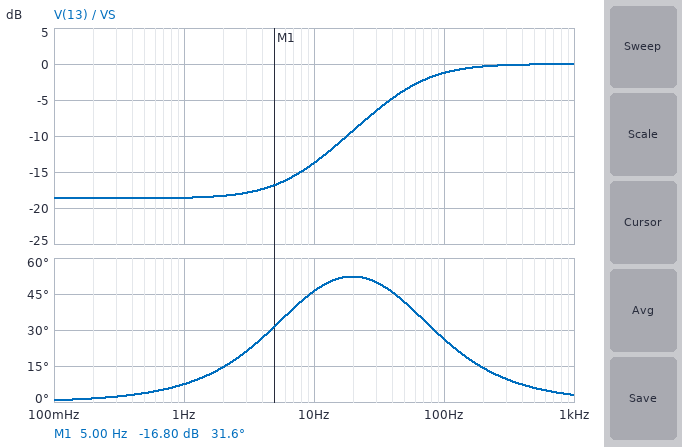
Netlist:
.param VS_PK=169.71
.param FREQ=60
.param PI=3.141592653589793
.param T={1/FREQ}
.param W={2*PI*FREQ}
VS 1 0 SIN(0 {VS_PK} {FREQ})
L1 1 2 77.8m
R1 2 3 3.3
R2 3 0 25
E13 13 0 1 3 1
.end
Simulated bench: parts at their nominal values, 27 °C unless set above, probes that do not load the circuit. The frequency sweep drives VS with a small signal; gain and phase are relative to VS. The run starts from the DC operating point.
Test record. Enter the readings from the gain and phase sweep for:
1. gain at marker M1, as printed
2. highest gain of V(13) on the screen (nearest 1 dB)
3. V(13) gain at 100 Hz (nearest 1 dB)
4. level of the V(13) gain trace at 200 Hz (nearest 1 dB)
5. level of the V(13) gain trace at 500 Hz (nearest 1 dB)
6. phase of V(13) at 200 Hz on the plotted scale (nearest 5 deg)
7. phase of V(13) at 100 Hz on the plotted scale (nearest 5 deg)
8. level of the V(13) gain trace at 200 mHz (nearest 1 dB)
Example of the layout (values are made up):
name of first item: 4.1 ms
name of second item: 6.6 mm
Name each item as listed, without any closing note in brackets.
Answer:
gain at marker M1, as printed: -16.80 dB
highest gain of V(13) on the screen: 0 dB
V(13) gain at 100 Hz: -1 dB
level of the V(13) gain trace at 200 Hz: 0 dB
level of the V(13) gain trace at 500 Hz: 0 dB
phase of V(13) at 200 Hz on the plotted scale: 15 deg
phase of V(13) at 100 Hz on the plotted scale: 25 deg
level of the V(13) gain trace at 200 mHz: -19 dB
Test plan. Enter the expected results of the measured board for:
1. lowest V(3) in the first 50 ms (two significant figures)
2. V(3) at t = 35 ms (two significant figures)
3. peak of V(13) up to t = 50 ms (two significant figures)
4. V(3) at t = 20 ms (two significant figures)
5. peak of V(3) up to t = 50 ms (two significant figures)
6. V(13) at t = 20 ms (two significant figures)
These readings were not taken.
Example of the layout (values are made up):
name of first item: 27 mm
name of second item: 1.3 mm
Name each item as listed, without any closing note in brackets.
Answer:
lowest V(3) in the first 50 ms: -100 V
V(3) at t = 35 ms: -18 V
peak of V(13) up to t = 50 ms: 120 V
V(3) at t = 20 ms: 46 V
peak of V(3) up to t = 50 ms: 110 V
V(13) at t = 20 ms: 120 V
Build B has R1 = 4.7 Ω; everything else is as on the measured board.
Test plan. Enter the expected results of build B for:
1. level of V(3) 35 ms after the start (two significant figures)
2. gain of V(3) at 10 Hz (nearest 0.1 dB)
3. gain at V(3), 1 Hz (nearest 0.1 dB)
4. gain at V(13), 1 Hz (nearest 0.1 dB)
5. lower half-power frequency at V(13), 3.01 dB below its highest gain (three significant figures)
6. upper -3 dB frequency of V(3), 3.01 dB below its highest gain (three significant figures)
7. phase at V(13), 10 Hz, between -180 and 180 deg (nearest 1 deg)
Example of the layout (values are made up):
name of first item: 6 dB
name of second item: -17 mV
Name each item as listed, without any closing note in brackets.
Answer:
level of V(3) 35 ms after the start: -15 V
gain of V(3) at 10 Hz: -1.6 dB
gain at V(3), 1 Hz: -1.5 dB
gain at V(13), 1 Hz: -16.0 dB
lower half-power frequency at V(13), 3.01 dB below its highest gain: 59.2 Hz
upper -3 dB frequency of V(3), 3.01 dB below its highest gain: 60.8 Hz
phase at V(13), 10 Hz, between -180 and 180 deg: 37 deg
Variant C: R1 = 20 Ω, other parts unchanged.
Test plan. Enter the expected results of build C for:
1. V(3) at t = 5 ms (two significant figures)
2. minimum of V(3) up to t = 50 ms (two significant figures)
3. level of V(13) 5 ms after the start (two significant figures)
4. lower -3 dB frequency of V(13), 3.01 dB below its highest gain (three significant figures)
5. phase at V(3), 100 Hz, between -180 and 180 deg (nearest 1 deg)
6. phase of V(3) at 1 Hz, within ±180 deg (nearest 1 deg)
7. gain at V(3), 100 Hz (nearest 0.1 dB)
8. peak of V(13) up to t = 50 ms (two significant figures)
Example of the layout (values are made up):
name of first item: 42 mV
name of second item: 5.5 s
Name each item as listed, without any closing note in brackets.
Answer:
V(3) at t = 5 ms: 79 V
minimum of V(3) up to t = 50 ms: -79 V
level of V(13) 5 ms after the start: 83 V
lower -3 dB frequency of V(13), 3.01 dB below its highest gain: 71.6 Hz
phase at V(3), 100 Hz, between -180 and 180 deg: -47 deg
phase of V(3) at 1 Hz, within ±180 deg: -1 deg
gain at V(3), 100 Hz: -8.5 dB
peak of V(13) up to t = 50 ms: 110 V
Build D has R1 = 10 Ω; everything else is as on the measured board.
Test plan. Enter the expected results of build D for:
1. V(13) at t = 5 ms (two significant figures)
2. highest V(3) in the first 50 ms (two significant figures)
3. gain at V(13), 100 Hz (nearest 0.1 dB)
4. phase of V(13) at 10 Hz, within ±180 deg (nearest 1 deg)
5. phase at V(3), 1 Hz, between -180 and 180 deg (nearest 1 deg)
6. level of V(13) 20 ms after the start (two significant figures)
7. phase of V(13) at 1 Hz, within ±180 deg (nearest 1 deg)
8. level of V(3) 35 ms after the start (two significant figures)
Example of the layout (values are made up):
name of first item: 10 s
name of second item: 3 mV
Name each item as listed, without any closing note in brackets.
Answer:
V(13) at t = 5 ms: 69 V
highest V(3) in the first 50 ms: 97 V
gain at V(13), 100 Hz: -1.6 dB
phase of V(13) at 10 Hz, within ±180 deg: 18 deg
phase at V(3), 1 Hz, between -180 and 180 deg: -1 deg
level of V(13) 20 ms after the start: 110 V
phase of V(13) at 1 Hz, within ±180 deg: 2 deg
level of V(3) 35 ms after the start: -6.4 V
